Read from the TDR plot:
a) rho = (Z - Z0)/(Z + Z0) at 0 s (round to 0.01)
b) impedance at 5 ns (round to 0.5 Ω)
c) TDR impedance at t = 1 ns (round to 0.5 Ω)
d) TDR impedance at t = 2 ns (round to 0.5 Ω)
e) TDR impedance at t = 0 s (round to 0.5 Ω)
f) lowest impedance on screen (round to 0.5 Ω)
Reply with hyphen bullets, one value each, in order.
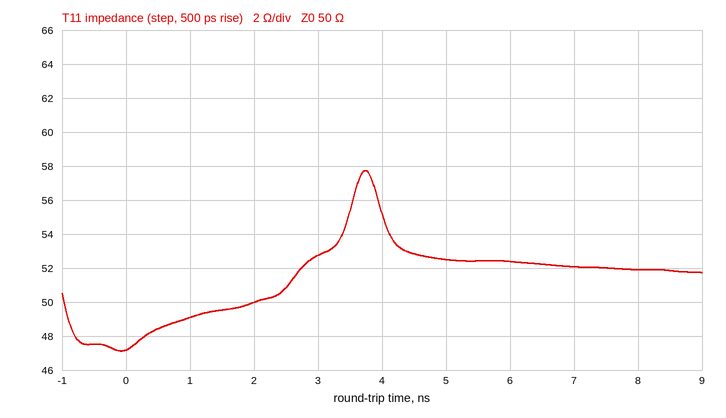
- -0.03
- 52.5 Ω
- 49.0 Ω
- 50.0 Ω
- 47.0 Ω
- 47.0 Ω
